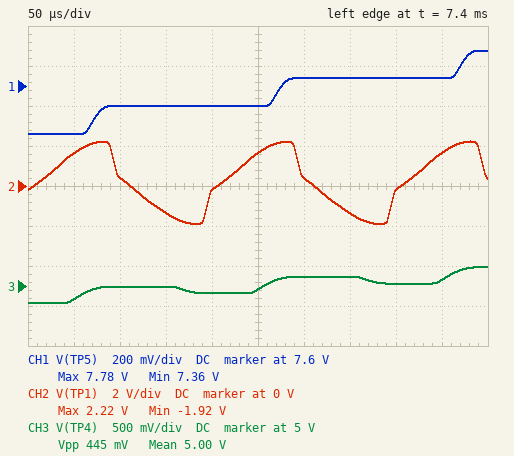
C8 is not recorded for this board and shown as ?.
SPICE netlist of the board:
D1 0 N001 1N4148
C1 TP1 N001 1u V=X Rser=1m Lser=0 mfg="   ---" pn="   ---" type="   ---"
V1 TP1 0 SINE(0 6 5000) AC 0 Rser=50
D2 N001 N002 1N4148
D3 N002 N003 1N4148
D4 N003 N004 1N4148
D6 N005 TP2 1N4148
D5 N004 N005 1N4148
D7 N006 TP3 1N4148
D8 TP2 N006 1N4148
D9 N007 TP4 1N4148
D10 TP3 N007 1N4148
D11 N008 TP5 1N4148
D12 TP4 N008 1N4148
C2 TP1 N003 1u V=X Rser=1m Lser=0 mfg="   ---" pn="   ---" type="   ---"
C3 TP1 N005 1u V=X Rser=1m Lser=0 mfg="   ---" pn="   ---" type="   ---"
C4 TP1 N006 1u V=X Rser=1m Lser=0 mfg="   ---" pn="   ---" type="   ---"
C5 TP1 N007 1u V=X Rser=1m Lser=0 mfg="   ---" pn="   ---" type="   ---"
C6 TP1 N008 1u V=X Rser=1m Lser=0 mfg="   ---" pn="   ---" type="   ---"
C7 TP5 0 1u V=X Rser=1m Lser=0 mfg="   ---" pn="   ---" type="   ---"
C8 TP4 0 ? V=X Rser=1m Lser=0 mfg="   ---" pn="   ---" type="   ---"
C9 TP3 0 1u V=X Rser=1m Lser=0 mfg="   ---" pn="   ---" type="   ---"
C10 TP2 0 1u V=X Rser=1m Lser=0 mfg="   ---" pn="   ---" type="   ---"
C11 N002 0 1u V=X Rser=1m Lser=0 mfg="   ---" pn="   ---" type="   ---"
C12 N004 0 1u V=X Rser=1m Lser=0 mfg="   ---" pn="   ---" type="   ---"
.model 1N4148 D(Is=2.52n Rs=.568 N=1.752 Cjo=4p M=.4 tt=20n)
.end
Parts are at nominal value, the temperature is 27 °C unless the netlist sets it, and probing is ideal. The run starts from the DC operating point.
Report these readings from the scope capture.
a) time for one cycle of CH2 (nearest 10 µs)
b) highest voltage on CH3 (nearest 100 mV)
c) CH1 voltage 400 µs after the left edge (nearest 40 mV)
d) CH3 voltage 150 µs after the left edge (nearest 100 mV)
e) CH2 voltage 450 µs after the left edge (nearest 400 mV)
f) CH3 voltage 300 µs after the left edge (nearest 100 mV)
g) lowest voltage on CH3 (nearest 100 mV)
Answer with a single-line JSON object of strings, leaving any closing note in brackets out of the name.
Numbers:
{"time for one cycle of CH2": "200 µs", "highest voltage on CH3": "5.2 V", "CH1 voltage 400 µs after the left edge": "7.64 V", "CH3 voltage 150 µs after the left edge": "5.0 V", "CH2 voltage 450 µs after the left edge": "1.6 V", "CH3 voltage 300 µs after the left edge": "5.1 V", "lowest voltage on CH3": "4.8 V"}
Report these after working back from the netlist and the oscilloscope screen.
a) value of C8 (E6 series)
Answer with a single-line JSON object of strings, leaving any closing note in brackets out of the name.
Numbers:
{"value of C8": "3.3 µF"}
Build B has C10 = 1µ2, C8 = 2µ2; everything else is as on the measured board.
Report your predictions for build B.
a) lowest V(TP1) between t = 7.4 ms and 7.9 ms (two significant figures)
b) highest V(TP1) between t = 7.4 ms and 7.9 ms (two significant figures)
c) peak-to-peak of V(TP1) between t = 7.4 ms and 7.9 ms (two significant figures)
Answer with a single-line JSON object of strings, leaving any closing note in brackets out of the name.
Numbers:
{"lowest V(TP1) between t = 7.4 ms and 7.9 ms": "-1.9 V", "highest V(TP1) between t = 7.4 ms and 7.9 ms": "2.3 V", "peak-to-peak of V(TP1) between t = 7.4 ms and 7.9 ms": "4.2 V"}
